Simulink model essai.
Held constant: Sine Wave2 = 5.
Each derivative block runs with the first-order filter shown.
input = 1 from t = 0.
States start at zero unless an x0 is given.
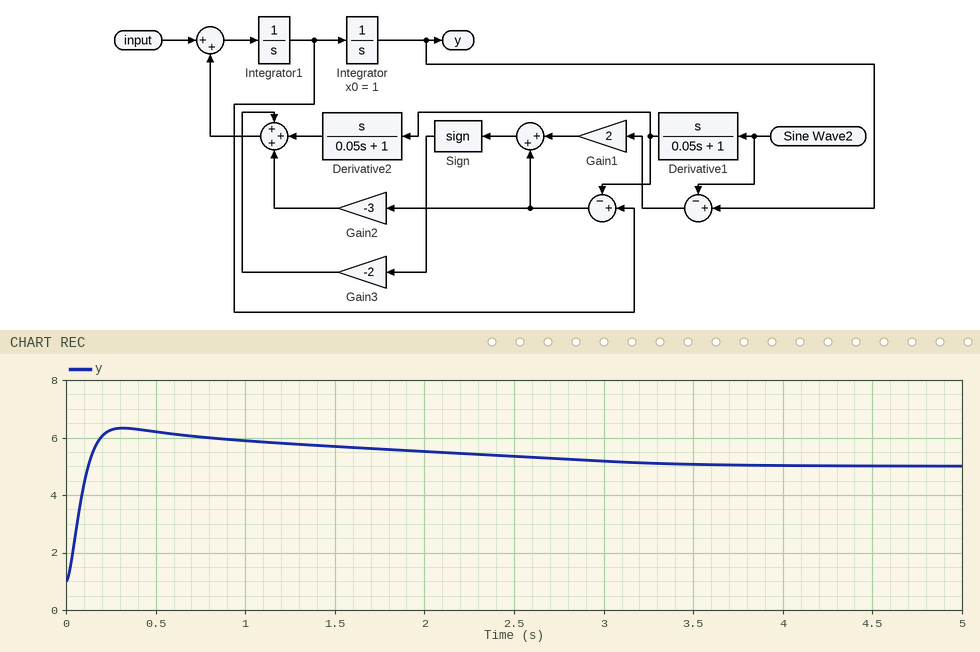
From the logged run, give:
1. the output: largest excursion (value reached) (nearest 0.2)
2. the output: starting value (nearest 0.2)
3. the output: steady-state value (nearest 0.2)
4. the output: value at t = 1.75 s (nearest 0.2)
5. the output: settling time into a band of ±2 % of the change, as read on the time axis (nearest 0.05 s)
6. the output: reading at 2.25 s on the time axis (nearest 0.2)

6.4
1.0
5.0
5.6
3.35 s
5.4
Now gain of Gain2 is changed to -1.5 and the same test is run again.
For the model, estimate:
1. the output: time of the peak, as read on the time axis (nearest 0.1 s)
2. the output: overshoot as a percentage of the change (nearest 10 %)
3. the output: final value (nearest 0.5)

0.4 s
30 %
5.0
